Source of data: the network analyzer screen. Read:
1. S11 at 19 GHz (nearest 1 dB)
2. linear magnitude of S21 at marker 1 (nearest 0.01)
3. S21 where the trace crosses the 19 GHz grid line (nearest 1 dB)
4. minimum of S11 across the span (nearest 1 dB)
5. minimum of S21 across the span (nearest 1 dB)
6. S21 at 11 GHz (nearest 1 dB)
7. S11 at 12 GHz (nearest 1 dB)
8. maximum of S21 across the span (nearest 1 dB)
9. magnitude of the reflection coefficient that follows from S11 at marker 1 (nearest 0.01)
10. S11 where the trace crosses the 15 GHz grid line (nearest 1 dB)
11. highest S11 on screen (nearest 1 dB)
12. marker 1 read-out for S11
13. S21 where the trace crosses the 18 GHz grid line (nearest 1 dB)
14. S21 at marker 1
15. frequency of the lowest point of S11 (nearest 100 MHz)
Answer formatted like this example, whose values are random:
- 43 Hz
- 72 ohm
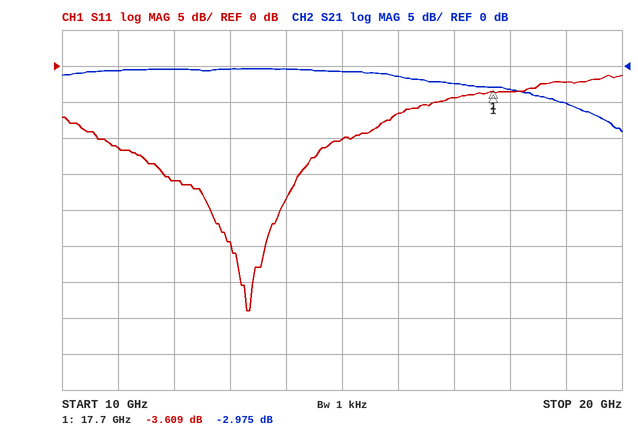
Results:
- -2 dB
- 0.71
- -5 dB
- -34 dB
- -9 dB
- -1 dB
- -16 dB
- 0 dB
- 0.66
- -10 dB
- -1 dB
- -3.609 dB
- -3 dB
- -2.975 dB
- 13.3 GHz
